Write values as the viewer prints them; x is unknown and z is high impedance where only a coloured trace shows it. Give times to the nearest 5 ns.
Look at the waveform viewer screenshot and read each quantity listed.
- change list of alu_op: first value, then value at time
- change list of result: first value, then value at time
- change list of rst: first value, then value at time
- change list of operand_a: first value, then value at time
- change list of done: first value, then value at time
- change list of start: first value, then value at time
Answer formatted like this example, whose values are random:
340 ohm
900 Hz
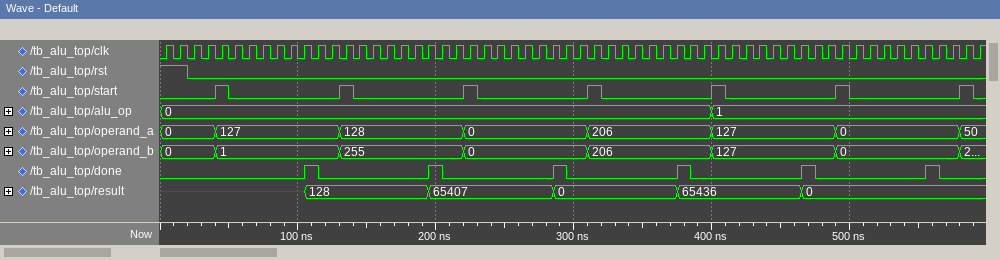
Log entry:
0, 1 at 400 ns
x, 128 at 105 ns, 65407 at 195 ns, 0 at 285 ns, 65436 at 375 ns, 0 at 465 ns
1, 0 at 20 ns
0, 127 at 40 ns, 128 at 130 ns, 0 at 220 ns, 206 at 310 ns, 127 at 400 ns, 0 at 490 ns, 50 at 580 ns
0, 1 at 105 ns, 0 at 115 ns, 1 at 195 ns, 0 at 205 ns, 1 at 285 ns, 0 at 295 ns, 1 at 375 ns, 0 at 385 ns, 1 at 465 ns, 0 at 475 ns, 1 at 555 ns, 0 at 565 ns
0, 1 at 40 ns, 0 at 50 ns, 1 at 130 ns, 0 at 140 ns, 1 at 220 ns, 0 at 230 ns, 1 at 310 ns, 0 at 320 ns, 1 at 400 ns, 0 at 410 ns, 1 at 490 ns, 0 at 500 ns, 1 at 580 ns, 0 at 590 ns
